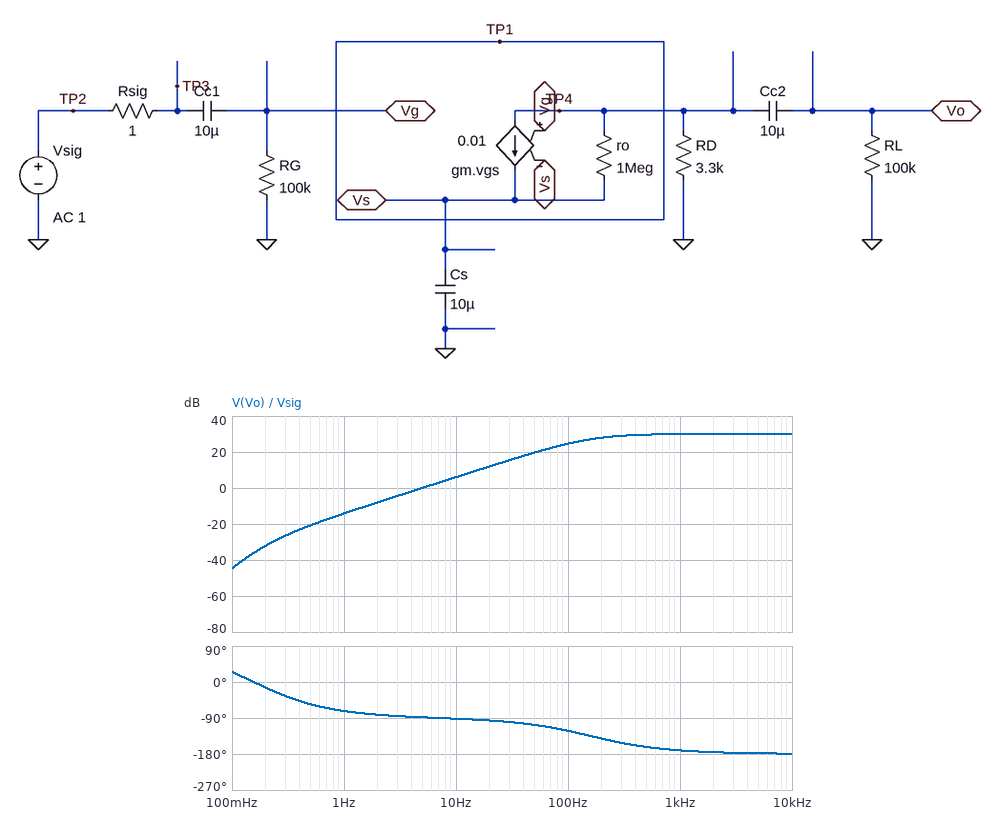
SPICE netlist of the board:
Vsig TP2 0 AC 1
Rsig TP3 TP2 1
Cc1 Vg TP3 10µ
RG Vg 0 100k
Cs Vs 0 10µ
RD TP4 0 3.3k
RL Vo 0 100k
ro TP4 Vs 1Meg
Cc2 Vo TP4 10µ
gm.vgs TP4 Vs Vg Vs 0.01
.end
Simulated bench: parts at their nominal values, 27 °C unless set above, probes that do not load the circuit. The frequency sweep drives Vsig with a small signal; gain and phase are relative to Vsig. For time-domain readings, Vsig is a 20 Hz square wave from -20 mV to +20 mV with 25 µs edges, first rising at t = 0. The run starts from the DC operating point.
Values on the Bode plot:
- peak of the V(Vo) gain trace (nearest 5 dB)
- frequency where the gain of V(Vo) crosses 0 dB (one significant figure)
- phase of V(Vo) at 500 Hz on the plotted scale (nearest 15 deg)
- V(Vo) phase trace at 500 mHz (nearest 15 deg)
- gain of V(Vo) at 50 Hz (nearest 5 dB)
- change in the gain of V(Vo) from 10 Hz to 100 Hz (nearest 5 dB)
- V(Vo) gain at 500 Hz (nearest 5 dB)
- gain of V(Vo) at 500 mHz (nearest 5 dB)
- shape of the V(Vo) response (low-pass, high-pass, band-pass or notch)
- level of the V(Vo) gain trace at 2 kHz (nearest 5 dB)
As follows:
30 dB
5 Hz
-165 deg
-60 deg
20 dB
20 dB
30 dB
-20 dB
high-pass
30 dB
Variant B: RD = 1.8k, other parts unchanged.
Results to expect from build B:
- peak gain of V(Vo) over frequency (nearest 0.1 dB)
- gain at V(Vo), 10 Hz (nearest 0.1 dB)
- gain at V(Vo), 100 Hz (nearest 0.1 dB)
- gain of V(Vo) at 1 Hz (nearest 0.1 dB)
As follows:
24.9 dB
0.9 dB
19.5 dB
-19.3 dB
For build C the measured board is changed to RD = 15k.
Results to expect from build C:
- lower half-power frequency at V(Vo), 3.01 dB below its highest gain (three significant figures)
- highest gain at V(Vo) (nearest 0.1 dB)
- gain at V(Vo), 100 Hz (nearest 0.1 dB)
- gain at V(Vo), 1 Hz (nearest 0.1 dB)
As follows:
157 Hz
42.2 dB
36.8 dB
-1.9 dB
